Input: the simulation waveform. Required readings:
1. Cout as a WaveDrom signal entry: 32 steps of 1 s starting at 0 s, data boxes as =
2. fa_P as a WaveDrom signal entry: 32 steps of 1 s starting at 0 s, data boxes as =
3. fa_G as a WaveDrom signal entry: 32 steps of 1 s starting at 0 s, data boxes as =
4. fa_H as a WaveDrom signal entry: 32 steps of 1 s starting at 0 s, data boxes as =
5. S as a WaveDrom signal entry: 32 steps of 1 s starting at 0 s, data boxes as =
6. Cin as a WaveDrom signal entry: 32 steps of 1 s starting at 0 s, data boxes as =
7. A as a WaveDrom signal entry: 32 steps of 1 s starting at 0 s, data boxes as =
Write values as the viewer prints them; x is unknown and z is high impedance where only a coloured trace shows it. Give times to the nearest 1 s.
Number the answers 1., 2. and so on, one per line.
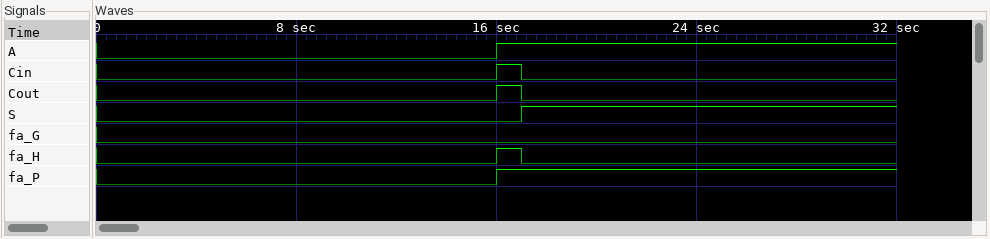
1. {name: 'Cout', wave: '0...............10..............'}
2. {name: 'fa_P', wave: '0...............1...............'}
3. {name: 'fa_G', wave: '0...............................'}
4. {name: 'fa_H', wave: '0...............10..............'}
5. {name: 'S', wave: '0................1..............'}
6. {name: 'Cin', wave: '0...............10..............'}
7. {name: 'A', wave: '0...............1...............'}
